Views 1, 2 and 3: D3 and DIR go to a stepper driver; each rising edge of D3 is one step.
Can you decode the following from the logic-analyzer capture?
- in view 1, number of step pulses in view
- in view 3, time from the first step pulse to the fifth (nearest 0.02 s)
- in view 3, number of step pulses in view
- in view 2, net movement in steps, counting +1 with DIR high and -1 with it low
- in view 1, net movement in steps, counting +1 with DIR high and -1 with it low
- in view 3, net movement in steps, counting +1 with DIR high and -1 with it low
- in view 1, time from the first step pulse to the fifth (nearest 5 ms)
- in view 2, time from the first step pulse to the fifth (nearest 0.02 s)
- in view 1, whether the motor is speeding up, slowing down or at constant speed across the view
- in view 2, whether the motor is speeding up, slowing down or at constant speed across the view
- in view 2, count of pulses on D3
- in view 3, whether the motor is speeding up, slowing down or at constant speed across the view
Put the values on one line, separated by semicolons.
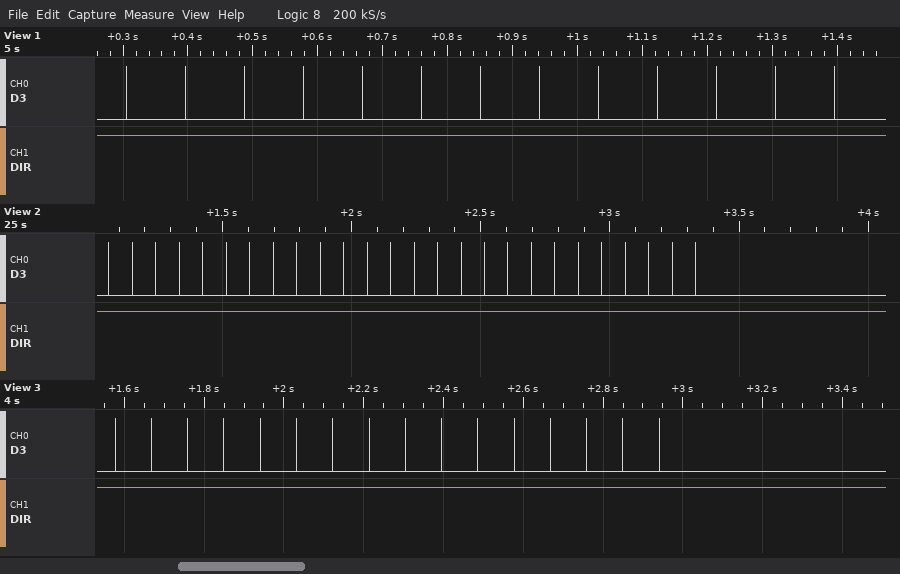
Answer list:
13; 0.36 s; 16; +26; +13; +16; 365 ms; 0.36 s; constant speed; constant speed; 26; constant speed
